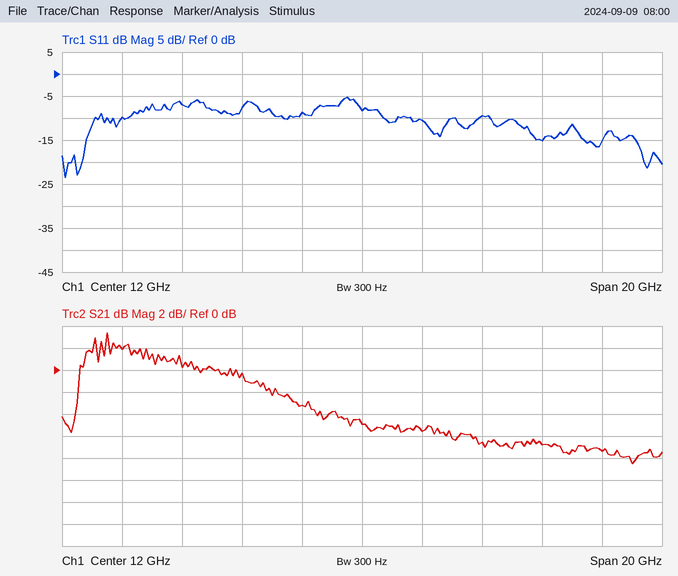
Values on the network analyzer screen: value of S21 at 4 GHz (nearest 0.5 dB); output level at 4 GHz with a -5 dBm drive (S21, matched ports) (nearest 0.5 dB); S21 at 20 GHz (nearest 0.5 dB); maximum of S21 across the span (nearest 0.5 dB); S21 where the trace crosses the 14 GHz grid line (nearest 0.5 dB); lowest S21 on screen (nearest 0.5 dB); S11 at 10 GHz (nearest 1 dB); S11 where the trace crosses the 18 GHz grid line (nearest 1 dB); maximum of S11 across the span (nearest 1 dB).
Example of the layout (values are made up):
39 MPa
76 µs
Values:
2.0 dB
-3.0 dBm
-7.5 dB
3.5 dB
-5.5 dB
-8.5 dB
-9 dB
-15 dB
-5 dB
